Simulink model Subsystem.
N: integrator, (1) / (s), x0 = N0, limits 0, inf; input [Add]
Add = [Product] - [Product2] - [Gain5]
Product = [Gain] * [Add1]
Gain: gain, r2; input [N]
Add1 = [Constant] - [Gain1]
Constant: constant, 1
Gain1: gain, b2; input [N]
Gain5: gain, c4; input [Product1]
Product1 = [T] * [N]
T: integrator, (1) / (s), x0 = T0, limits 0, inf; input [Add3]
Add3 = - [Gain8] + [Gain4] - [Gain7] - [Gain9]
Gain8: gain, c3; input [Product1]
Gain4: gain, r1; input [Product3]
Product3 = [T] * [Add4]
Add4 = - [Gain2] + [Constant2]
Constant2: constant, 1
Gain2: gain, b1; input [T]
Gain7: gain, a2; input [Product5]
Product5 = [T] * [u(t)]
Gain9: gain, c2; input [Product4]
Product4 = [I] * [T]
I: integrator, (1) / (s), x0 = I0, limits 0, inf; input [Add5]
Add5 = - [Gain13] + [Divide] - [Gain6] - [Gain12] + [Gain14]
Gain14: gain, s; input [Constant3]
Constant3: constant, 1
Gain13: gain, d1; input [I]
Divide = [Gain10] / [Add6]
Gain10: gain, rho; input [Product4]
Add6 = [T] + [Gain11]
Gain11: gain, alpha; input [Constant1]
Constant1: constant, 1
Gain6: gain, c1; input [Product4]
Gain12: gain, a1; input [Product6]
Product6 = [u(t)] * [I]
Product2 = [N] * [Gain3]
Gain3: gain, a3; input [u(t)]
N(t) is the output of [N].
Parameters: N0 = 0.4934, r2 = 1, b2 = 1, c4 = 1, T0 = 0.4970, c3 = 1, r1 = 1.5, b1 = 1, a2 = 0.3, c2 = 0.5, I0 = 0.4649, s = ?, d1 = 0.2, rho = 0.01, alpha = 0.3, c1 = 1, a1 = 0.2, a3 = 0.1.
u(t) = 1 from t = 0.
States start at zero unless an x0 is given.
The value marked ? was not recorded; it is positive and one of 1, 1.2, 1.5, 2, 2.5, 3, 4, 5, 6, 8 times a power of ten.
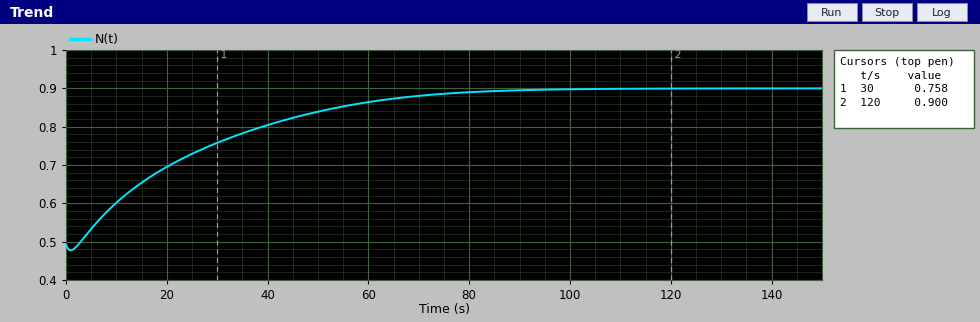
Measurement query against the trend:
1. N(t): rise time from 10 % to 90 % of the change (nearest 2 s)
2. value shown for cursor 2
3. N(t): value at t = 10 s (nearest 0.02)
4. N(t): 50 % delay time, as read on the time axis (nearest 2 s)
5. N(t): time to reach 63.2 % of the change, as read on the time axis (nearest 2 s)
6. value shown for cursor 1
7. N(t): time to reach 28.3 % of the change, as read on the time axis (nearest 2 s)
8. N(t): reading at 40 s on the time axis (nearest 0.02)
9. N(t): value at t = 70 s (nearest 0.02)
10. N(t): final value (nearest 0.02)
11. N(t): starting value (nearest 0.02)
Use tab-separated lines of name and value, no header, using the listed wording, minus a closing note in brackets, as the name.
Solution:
N(t): rise time from 10 % to 90 % of the change	52 s
value shown for cursor 2	0.900
N(t): value at t = 10 s	0.60
N(t): 50 % delay time, as read on the time axis	20 s
N(t): time to reach 63.2 % of the change, as read on the time axis	28 s
value shown for cursor 1	0.758
N(t): time to reach 28.3 % of the change, as read on the time axis	10 s
N(t): reading at 40 s on the time axis	0.80
N(t): value at t = 70 s	0.88
N(t): final value	0.90
N(t): starting value	0.50
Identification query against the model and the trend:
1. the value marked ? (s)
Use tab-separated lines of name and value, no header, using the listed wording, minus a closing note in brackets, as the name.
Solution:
the value marked ?	0.3
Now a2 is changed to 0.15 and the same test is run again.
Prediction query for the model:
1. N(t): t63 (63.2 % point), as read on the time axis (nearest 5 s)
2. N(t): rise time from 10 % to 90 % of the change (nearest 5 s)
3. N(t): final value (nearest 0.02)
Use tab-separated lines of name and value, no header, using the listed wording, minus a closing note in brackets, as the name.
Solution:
N(t): t63 (63.2 % point), as read on the time axis	15 s
N(t): rise time from 10 % to 90 % of the change	35 s
N(t): final value	0.30
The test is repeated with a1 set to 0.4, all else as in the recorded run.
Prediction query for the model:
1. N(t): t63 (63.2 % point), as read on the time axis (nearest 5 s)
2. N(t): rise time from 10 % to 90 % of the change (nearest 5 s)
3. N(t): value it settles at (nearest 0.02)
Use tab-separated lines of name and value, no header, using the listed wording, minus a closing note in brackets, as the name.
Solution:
N(t): t63 (63.2 % point), as read on the time axis	20 s
N(t): rise time from 10 % to 90 % of the change	40 s
N(t): value it settles at	0.66
